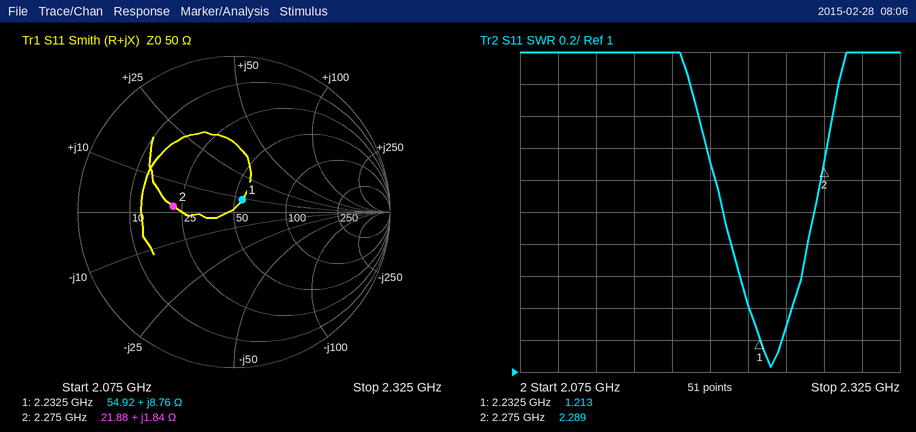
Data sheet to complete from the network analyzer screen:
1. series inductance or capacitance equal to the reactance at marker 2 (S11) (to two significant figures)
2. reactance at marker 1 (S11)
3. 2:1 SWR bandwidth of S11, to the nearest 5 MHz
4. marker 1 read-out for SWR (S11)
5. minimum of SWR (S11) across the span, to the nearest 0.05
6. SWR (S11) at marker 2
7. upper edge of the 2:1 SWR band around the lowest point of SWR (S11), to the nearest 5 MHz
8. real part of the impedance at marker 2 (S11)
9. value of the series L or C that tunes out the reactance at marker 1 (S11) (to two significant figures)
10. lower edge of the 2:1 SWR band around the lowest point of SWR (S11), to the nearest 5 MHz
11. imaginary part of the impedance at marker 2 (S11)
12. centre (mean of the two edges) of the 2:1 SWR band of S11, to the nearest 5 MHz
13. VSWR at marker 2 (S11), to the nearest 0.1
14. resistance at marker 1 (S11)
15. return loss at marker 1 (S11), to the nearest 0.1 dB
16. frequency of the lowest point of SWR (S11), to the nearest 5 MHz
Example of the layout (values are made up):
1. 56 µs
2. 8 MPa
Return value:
1. 130 pH
2. +8.76 Ω
3. 60 MHz
4. 1.213
5. 1.05
6. 2.289
7. 2.270 GHz
8. 21.88 Ω
9. 8.1 pF
10. 2.210 GHz
11. +1.84 Ω
12. 2.240 GHz
13. 2.3
14. 54.92 Ω
15. 20.4 dB
16. 2.240 GHz
